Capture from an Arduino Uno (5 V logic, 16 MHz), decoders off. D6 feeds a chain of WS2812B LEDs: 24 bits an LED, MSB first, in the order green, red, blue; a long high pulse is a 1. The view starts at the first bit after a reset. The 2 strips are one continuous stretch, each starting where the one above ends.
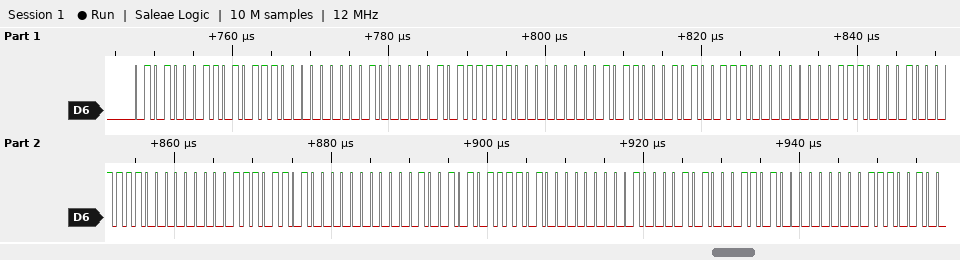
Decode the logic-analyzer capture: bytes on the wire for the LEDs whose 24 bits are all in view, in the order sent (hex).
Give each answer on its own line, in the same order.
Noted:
51 AE 00 81 7E 00 B1 4E 00 E1 1E 00 ED 00 12 BD 00 42 8D 00 72
